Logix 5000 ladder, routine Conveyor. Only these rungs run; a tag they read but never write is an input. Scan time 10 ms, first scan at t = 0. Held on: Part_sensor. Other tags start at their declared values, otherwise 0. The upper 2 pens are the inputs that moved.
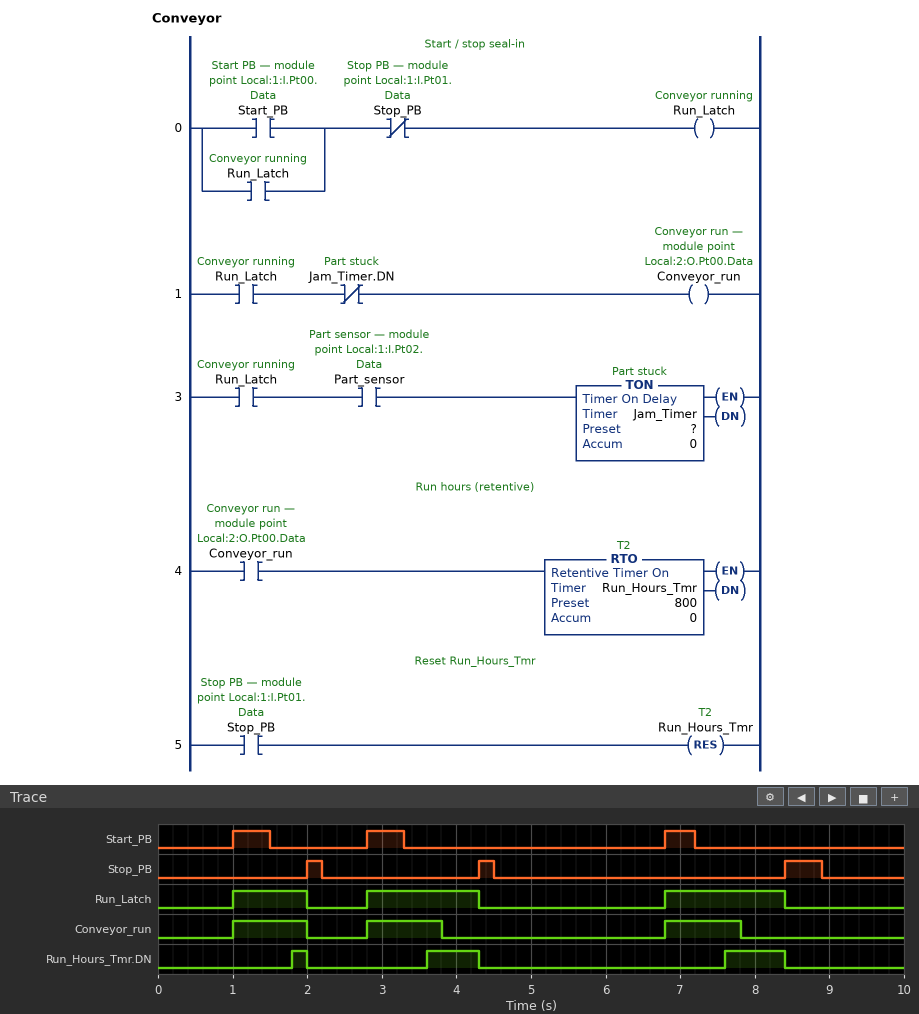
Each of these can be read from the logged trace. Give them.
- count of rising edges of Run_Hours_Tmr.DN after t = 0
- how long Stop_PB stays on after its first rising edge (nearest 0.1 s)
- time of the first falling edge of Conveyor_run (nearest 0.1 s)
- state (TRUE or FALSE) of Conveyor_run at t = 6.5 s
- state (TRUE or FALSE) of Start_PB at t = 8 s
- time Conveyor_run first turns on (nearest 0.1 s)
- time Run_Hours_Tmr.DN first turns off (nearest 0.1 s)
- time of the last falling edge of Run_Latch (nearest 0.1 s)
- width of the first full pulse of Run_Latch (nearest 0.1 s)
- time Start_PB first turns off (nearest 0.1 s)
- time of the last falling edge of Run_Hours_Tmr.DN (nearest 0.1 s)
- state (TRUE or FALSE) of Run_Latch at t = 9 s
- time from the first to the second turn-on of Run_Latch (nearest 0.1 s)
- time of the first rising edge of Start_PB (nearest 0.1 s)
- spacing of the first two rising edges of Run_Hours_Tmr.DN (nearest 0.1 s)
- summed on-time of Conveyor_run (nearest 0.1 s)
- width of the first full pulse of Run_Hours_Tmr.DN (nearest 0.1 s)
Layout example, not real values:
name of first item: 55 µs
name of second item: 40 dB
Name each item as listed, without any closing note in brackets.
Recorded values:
count of rising edges of Run_Hours_Tmr.DN after t = 0: 3
how long Stop_PB stays on after its first rising edge: 0.2 s
time of the first falling edge of Conveyor_run: 2.0 s
state (TRUE or FALSE) of Conveyor_run at t = 6.5 s: FALSE
state (TRUE or FALSE) of Start_PB at t = 8 s: FALSE
time Conveyor_run first turns on: 1.0 s
time Run_Hours_Tmr.DN first turns off: 2.0 s
time of the last falling edge of Run_Latch: 8.4 s
width of the first full pulse of Run_Latch: 1.0 s
time Start_PB first turns off: 1.5 s
time of the last falling edge of Run_Hours_Tmr.DN: 8.4 s
state (TRUE or FALSE) of Run_Latch at t = 9 s: FALSE
time from the first to the second turn-on of Run_Latch: 1.8 s
time of the first rising edge of Start_PB: 1.0 s
spacing of the first two rising edges of Run_Hours_Tmr.DN: 1.8 s
summed on-time of Conveyor_run: 3.0 s
width of the first full pulse of Run_Hours_Tmr.DN: 0.2 s
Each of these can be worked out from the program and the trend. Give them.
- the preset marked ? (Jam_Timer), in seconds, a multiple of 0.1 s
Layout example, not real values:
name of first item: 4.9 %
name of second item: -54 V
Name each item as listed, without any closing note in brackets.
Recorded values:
the preset marked ? (Jam_Timer), in seconds, a multiple of 0.1 s: 1.0 s
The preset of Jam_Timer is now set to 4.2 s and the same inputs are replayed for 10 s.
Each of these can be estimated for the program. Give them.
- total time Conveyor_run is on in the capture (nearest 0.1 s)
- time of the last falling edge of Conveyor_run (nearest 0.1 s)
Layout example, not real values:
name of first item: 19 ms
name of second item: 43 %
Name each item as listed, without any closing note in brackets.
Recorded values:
total time Conveyor_run is on in the capture: 4.1 s
time of the last falling edge of Conveyor_run: 8.4 s
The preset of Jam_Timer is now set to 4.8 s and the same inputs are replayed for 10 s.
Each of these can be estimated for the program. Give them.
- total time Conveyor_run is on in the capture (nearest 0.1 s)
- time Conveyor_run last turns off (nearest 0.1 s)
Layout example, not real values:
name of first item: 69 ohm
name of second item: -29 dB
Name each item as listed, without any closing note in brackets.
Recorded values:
total time Conveyor_run is on in the capture: 4.1 s
time Conveyor_run last turns off: 8.4 s
